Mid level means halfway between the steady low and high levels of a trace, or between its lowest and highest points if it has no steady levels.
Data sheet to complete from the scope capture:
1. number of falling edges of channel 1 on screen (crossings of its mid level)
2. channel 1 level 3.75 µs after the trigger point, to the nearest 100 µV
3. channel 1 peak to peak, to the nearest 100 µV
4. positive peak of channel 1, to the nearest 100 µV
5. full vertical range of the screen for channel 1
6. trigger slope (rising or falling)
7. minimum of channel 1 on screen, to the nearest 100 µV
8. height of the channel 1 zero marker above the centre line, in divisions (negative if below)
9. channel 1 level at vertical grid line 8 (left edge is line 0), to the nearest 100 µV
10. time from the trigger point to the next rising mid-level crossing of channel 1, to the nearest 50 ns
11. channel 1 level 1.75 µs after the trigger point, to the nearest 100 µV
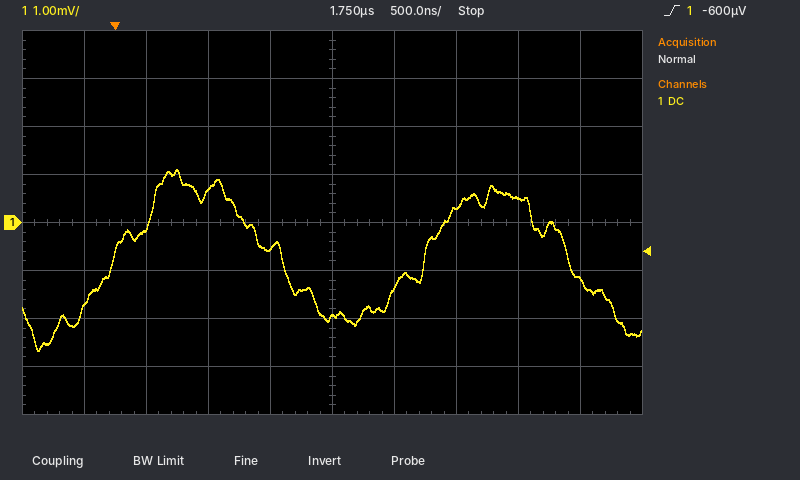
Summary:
2
-1.2 mV
3.8 mV
1.1 mV
8 mV
rising
-2.7 mV
0.0 div
500 µV
2.50 µs
-2.0 mV
